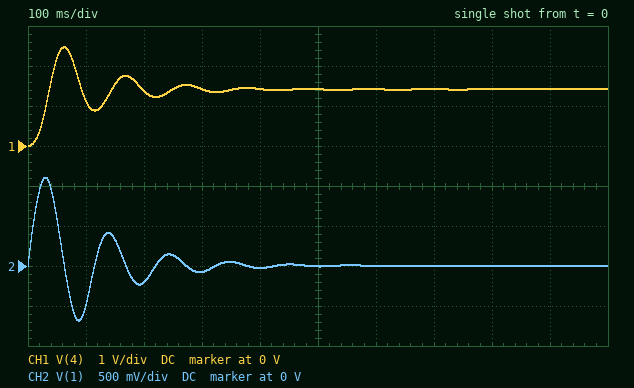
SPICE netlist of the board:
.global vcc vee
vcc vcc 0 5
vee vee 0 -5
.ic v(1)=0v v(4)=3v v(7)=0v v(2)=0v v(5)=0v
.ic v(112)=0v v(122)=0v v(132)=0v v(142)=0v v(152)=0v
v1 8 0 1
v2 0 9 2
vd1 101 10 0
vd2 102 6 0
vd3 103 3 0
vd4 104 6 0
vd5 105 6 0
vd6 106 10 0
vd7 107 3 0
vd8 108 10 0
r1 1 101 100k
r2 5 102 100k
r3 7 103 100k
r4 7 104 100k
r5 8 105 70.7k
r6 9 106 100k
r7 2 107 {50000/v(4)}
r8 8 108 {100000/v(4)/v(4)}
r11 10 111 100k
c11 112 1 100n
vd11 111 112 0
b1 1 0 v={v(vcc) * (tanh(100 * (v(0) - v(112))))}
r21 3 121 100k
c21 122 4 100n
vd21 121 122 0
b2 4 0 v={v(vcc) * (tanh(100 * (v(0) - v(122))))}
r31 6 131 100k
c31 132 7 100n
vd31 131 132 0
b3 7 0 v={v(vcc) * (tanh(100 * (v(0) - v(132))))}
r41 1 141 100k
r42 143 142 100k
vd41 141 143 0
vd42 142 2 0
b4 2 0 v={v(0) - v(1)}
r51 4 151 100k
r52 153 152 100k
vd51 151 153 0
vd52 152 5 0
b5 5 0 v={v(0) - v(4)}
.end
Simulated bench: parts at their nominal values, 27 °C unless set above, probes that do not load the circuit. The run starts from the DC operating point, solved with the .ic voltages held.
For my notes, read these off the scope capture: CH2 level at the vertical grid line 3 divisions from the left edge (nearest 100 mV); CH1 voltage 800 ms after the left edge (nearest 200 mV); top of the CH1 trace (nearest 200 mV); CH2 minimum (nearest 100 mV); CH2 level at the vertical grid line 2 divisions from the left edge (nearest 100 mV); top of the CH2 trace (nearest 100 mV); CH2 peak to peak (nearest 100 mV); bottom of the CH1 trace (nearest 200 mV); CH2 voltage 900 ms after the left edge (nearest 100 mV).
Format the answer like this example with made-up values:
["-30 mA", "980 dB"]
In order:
["-100 mV", "1.4 V", "2.4 V", "-700 mV", "-200 mV", "1.1 V", "1.8 V", "0 V", "0 V"]
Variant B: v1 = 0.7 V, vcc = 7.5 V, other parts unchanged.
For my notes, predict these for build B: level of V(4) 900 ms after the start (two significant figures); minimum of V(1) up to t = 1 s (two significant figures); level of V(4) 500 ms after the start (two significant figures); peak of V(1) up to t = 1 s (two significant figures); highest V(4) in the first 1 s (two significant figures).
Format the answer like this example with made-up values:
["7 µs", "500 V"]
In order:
["1.6 V", "-570 mV", "1.5 V", "1.2 V", "3.0 V"]
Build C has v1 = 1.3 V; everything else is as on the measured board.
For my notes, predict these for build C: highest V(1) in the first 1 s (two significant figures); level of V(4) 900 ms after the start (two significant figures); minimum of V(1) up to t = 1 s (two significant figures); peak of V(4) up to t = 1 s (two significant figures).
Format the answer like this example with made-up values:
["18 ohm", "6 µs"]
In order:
["1.0 V", "1.3 V", "-810 mV", "2.2 V"]
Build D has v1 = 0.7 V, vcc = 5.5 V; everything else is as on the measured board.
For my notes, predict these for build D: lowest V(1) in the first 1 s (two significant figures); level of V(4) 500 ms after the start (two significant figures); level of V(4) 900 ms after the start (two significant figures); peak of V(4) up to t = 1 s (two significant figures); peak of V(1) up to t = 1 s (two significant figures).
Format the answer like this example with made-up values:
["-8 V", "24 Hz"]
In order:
["-570 mV", "1.5 V", "1.6 V", "3.0 V", "1.2 V"]
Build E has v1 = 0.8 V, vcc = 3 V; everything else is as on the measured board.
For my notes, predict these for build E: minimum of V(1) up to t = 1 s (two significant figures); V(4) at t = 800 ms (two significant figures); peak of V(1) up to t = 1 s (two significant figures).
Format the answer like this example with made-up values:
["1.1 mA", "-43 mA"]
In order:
["-590 mV", "1.5 V", "1.2 V"]
